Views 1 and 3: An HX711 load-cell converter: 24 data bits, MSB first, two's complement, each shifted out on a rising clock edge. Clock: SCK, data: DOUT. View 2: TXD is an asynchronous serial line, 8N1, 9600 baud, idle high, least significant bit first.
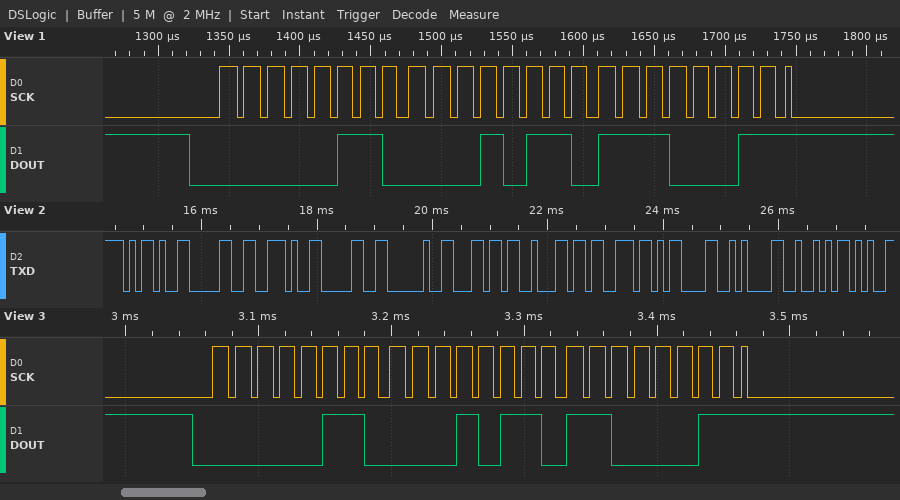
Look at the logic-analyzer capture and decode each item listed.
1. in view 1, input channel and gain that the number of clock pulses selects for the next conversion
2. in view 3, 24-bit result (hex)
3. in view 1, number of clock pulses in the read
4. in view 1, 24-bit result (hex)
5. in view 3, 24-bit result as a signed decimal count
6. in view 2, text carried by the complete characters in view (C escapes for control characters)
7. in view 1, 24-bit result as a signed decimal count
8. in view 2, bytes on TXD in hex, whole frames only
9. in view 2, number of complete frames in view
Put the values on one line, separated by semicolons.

channel A, gain 128; 0x0616C3; 25; 0x0616E3; 399043; "-0.0 lbs\r\nR"; 399075; 2D 30 2E 30 20 6C 62 73 0D 0A 52; 11
